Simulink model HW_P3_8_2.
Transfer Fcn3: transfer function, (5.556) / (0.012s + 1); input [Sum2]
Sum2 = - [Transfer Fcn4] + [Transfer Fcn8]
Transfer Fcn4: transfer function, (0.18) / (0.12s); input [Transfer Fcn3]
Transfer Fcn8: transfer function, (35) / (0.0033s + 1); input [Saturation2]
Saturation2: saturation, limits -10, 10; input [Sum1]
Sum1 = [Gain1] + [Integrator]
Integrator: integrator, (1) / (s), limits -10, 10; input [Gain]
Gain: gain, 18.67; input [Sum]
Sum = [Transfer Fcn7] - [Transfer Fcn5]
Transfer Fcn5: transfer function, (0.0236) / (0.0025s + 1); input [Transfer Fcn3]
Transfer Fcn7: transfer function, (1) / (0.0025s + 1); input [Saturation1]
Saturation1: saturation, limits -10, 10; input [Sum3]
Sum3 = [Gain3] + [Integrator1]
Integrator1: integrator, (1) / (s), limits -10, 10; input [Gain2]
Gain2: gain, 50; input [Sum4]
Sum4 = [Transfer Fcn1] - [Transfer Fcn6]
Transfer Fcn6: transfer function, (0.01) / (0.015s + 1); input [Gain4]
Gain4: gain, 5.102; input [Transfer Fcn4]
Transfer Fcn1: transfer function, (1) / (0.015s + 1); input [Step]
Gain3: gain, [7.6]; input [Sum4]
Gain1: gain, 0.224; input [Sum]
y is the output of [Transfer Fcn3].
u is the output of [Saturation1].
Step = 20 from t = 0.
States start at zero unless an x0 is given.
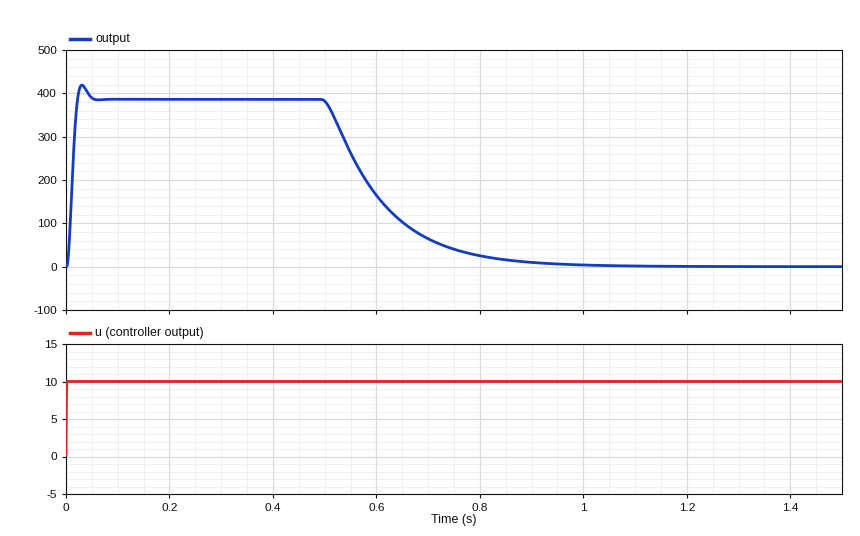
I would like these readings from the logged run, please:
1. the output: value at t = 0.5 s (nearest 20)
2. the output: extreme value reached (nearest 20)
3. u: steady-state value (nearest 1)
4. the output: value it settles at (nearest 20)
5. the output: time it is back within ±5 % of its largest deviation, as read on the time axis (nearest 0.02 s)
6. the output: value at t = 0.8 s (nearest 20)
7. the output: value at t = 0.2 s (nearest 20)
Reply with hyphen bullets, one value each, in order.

- 380
- 420
- 10
- 0
- 0.82 s
- 20
- 380
